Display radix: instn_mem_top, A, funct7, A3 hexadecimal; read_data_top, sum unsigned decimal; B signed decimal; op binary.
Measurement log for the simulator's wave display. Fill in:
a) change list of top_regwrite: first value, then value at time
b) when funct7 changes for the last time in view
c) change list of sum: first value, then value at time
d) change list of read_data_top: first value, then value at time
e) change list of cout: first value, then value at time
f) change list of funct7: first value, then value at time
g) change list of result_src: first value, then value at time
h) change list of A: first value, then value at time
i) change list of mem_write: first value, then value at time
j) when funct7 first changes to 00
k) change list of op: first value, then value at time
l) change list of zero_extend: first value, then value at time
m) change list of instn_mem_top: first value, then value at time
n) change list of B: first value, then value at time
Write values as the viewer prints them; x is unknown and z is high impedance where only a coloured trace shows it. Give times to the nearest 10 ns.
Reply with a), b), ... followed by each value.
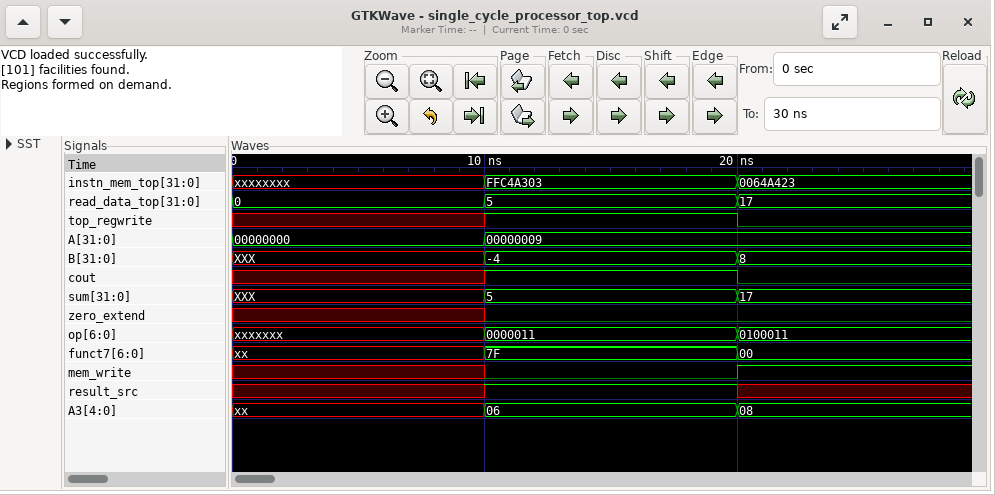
a) x, 1 at 10 ns, 0 at 20 ns
b) 20 ns
c) XXX, 5 at 10 ns, 17 at 20 ns
d) 0, 5 at 10 ns, 17 at 20 ns
e) x, 1 at 10 ns, 0 at 20 ns
f) xx, 7F at 10 ns, 00 at 20 ns
g) x, 1 at 10 ns, x at 20 ns
h) 00000000, 00000009 at 10 ns
i) x, 0 at 10 ns, 1 at 20 ns
j) 20 ns
k) xxxxxxx, 0000011 at 10 ns, 0100011 at 20 ns
l) x, 0 at 10 ns
m) xxxxxxxx, FFC4A303 at 10 ns, 0064A423 at 20 ns
n) XXX, -4 at 10 ns, 8 at 20 ns
